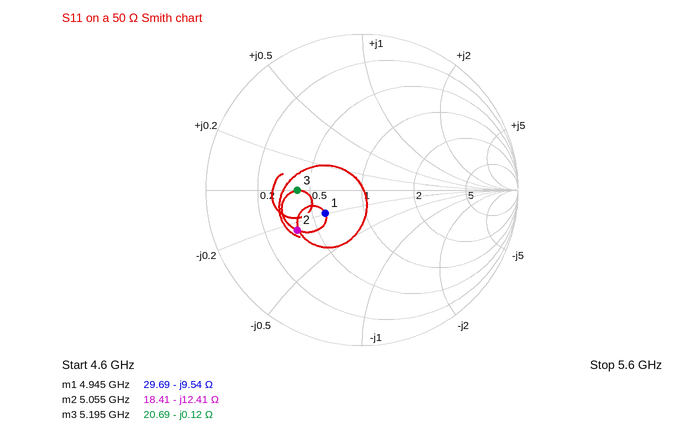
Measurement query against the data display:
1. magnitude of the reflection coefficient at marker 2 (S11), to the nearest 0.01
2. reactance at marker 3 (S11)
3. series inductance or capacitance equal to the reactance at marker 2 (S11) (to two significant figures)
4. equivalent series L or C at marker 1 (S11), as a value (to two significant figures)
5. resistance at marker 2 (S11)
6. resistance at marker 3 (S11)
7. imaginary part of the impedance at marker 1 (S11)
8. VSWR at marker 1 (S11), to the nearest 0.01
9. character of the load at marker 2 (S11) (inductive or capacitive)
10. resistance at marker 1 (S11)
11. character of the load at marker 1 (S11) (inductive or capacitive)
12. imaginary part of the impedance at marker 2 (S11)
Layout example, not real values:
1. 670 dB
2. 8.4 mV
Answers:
1. 0.49
2. -0.12 Ω
3. 2.5 pF
4. 3.4 pF
5. 18.41 Ω
6. 20.69 Ω
7. -9.54 Ω
8. 1.78
9. capacitive
10. 29.69 Ω
11. capacitive
12. -12.41 Ω
